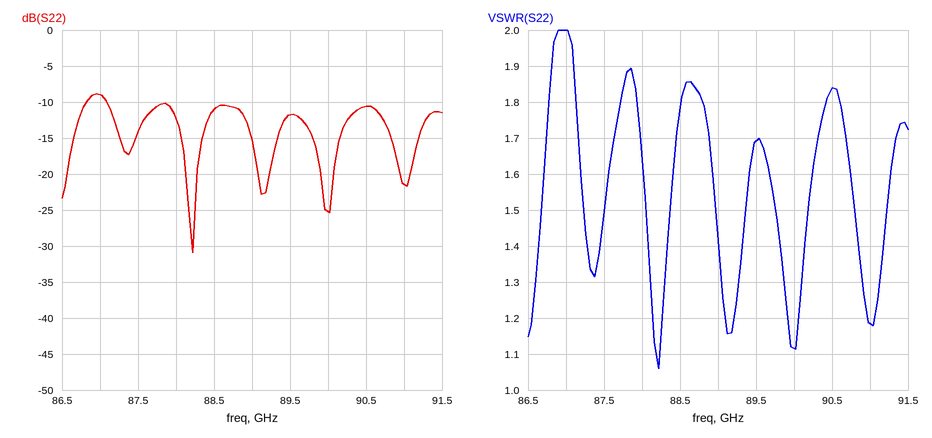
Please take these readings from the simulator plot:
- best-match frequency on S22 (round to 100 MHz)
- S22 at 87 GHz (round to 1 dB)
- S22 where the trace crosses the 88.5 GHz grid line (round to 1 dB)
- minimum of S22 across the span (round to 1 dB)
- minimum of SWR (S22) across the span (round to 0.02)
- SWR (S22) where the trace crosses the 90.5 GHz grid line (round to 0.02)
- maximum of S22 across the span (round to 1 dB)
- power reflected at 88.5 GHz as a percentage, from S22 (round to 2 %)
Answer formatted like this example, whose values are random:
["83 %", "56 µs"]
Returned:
["88.2 GHz", "-9 dB", "-11 dB", "-31 dB", "1.06", "1.84", "-9 dB", "8 %"]
